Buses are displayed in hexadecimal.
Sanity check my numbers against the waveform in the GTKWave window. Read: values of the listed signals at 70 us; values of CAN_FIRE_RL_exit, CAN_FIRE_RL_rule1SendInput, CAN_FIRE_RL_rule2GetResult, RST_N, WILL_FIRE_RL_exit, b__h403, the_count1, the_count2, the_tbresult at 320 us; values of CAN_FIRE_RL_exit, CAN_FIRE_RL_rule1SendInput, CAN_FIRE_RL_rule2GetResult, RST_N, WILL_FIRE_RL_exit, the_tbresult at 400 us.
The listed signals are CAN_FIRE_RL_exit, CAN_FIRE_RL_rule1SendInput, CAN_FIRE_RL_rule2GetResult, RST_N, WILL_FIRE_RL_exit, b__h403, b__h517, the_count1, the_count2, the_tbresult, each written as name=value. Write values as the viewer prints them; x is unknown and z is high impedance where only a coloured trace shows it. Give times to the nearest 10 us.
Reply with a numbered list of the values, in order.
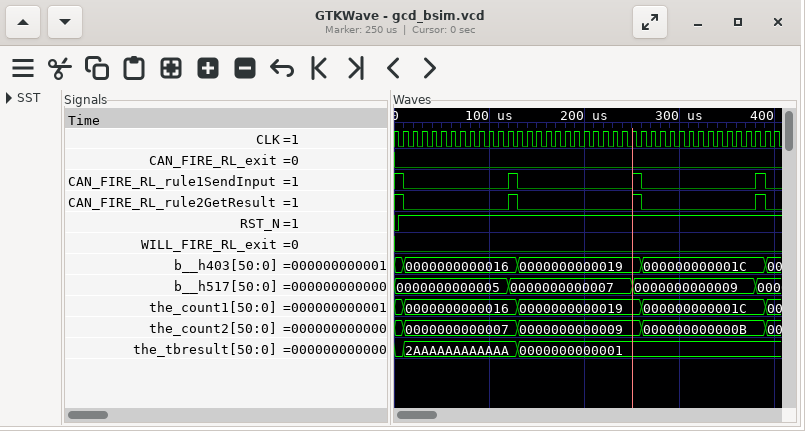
1. CAN_FIRE_RL_exit=0, CAN_FIRE_RL_rule1SendInput=0, CAN_FIRE_RL_rule2GetResult=0, RST_N=1, WILL_FIRE_RL_exit=0, b__h403=0000000000016, b__h517=0000000000005, the_count1=0000000000016, the_count2=0000000000007, the_tbresult=2AAAAAAAAAAAA
2. CAN_FIRE_RL_exit=0, CAN_FIRE_RL_rule1SendInput=0, CAN_FIRE_RL_rule2GetResult=0, RST_N=1, WILL_FIRE_RL_exit=0, b__h403=000000000001C, the_count1=000000000001C, the_count2=000000000000B, the_tbresult=0000000000001
3. CAN_FIRE_RL_exit=0, CAN_FIRE_RL_rule1SendInput=0, CAN_FIRE_RL_rule2GetResult=0, RST_N=1, WILL_FIRE_RL_exit=0, the_tbresult=0000000000001
